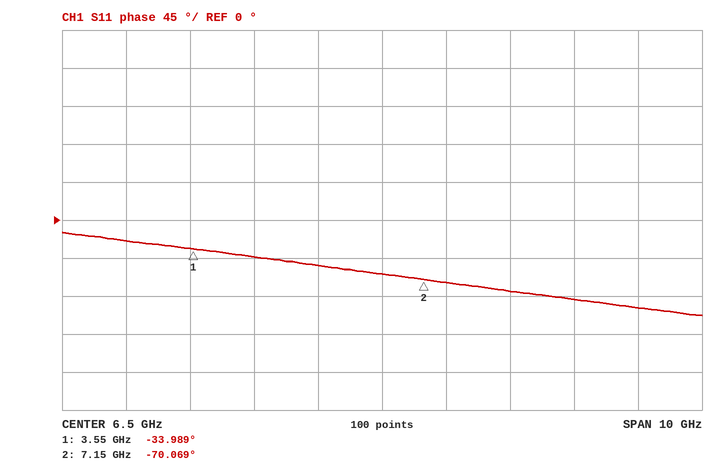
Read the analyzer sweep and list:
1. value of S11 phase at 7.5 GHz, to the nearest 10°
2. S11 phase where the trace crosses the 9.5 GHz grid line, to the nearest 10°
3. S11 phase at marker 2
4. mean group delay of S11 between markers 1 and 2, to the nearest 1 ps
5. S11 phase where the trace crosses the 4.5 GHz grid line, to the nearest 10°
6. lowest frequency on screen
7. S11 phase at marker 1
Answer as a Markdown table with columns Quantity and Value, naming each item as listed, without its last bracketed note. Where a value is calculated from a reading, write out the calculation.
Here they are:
| Quantity | Value |
|---|---|
| value of S11 phase at 7.5 GHz, to the nearest 10° | -70° |
| S11 phase where the trace crosses the 9.5 GHz grid line, to the nearest 10° | -90° |
| S11 phase at marker 2 | -70.069° |
| mean group delay of S11 between markers 1 and 2, to the nearest 1 ps | −(-70.069° − (-33.989°))/(360° × 3.6 GHz) ≈ 28 ps |
| S11 phase where the trace crosses the 4.5 GHz grid line, to the nearest 10° | -40° |
| lowest frequency on screen | 1.5 GHz |
| S11 phase at marker 1 | -33.989° |
